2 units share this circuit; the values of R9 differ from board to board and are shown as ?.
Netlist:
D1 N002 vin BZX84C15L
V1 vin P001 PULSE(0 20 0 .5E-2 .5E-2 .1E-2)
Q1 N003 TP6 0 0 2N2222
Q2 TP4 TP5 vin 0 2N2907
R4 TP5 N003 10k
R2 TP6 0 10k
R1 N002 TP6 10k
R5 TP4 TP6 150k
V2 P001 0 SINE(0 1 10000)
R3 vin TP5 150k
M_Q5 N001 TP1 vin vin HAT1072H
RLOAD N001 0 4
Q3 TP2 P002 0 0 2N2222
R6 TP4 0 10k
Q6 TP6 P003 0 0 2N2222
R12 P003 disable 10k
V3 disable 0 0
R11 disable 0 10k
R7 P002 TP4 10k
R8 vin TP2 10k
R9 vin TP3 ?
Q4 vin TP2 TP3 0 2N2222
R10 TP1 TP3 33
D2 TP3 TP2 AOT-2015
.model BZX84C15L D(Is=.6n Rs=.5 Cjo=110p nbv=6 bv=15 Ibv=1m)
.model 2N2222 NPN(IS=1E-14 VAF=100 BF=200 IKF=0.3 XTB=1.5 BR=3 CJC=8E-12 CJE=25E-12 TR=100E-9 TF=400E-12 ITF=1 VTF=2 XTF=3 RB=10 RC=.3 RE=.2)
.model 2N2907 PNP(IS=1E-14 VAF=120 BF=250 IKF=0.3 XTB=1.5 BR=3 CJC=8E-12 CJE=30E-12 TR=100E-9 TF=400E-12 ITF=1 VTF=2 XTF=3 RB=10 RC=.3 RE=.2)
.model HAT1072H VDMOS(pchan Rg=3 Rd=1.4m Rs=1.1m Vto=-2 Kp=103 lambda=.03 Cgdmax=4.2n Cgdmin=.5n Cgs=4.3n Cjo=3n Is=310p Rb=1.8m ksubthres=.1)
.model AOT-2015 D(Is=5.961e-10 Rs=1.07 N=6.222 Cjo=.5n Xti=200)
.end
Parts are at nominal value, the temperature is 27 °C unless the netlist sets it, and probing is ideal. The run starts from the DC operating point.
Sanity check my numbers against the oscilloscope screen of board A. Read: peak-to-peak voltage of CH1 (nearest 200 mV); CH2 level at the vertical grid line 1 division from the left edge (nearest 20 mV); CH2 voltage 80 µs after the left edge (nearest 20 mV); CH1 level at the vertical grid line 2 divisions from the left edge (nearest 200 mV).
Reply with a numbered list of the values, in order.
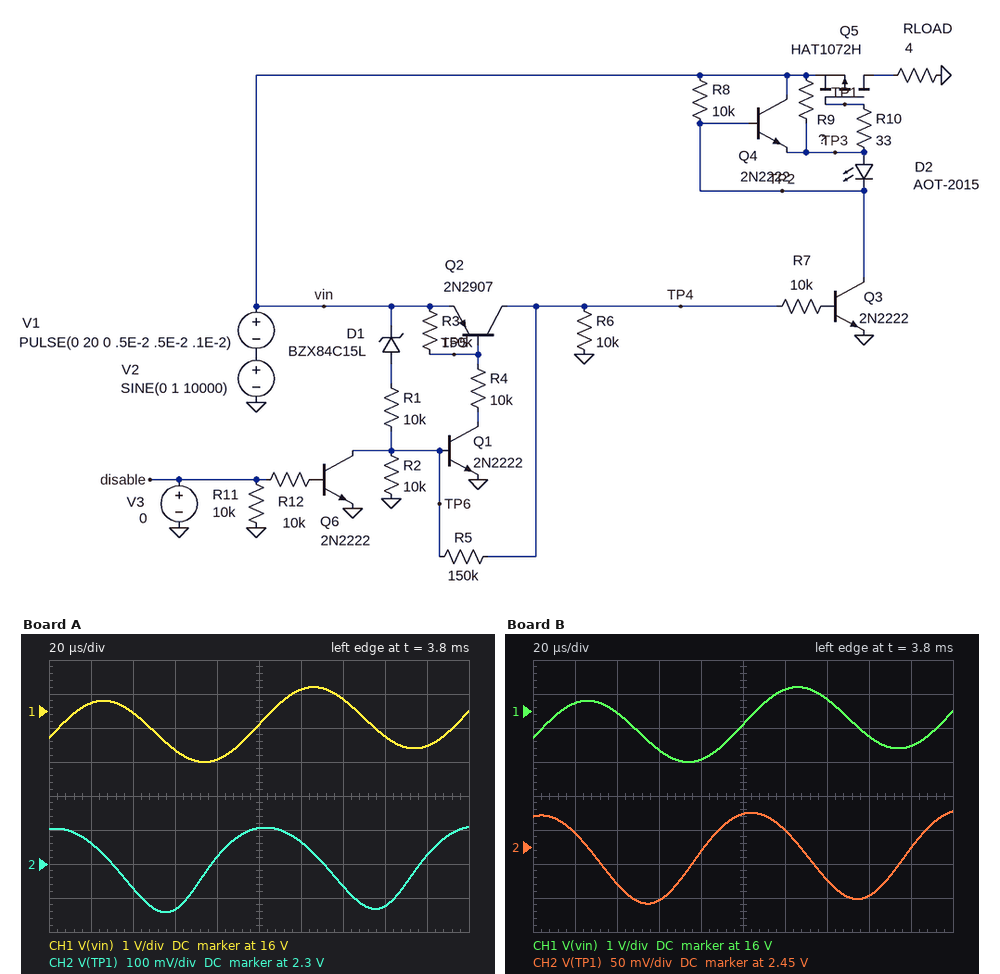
1. 2.2 V
2. 2.36 V
3. 2.32 V
4. 16.0 V
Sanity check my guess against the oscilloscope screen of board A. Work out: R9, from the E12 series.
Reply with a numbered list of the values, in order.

1. 15 kΩ
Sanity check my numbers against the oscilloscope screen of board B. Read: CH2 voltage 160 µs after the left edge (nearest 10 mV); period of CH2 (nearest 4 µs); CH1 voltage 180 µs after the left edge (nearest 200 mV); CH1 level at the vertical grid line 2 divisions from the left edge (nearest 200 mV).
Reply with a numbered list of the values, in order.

1. 2.38 V
2. 100 µs
3. 15.0 V
4. 16.0 V
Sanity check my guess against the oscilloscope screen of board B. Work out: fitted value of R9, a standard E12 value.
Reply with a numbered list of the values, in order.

1. 6.8 kΩ
